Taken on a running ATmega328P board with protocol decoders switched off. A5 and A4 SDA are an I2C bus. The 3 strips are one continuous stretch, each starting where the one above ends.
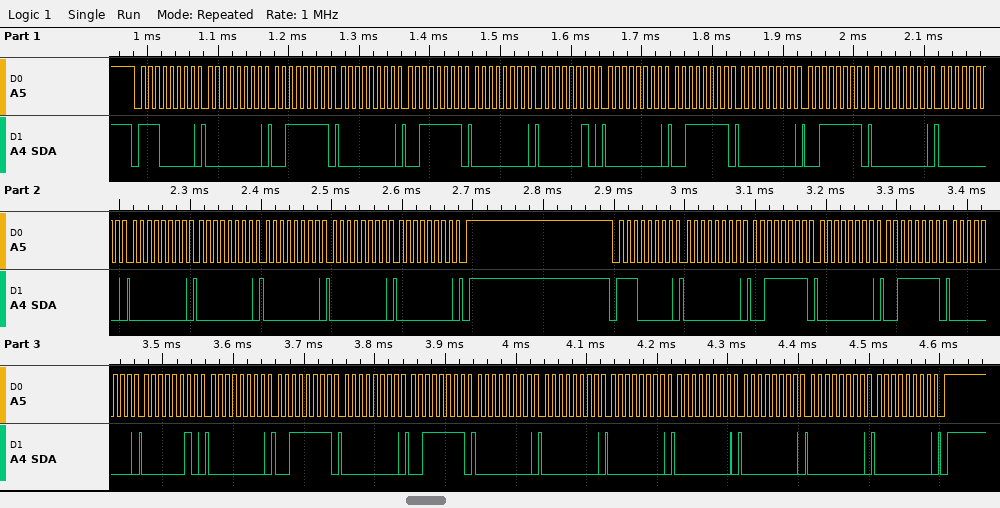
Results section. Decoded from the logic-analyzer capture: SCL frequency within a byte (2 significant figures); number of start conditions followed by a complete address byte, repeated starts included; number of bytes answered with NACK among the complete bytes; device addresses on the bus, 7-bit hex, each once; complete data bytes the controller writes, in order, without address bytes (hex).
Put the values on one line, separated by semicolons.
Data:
100 kHz; 2; 0; 0x70; 00 3F 00 3F 00 02 00 3F 00 3F 00 00 00 00 00 00 00 00 3F 00 3F 00 02 00 3F 00 3F 00 00 00 00 00 00 00
